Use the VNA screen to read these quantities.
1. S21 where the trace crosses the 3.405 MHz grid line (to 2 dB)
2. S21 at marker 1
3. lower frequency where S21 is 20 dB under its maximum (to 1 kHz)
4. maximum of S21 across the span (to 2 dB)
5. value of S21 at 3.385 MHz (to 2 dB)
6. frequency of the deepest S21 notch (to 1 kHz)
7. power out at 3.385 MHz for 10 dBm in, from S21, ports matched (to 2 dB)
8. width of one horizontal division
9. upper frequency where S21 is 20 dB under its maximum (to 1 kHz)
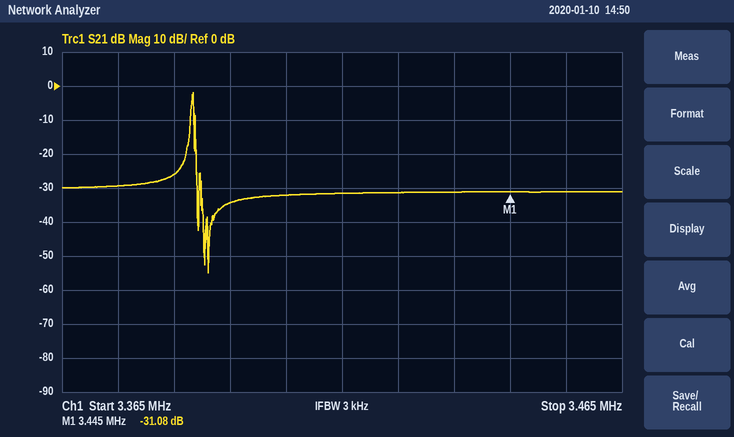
-32 dB
-31.08 dB
3.387 MHz
-2 dB
-26 dB
3.391 MHz
-16 dBm
10 kHz
3.389 MHz
